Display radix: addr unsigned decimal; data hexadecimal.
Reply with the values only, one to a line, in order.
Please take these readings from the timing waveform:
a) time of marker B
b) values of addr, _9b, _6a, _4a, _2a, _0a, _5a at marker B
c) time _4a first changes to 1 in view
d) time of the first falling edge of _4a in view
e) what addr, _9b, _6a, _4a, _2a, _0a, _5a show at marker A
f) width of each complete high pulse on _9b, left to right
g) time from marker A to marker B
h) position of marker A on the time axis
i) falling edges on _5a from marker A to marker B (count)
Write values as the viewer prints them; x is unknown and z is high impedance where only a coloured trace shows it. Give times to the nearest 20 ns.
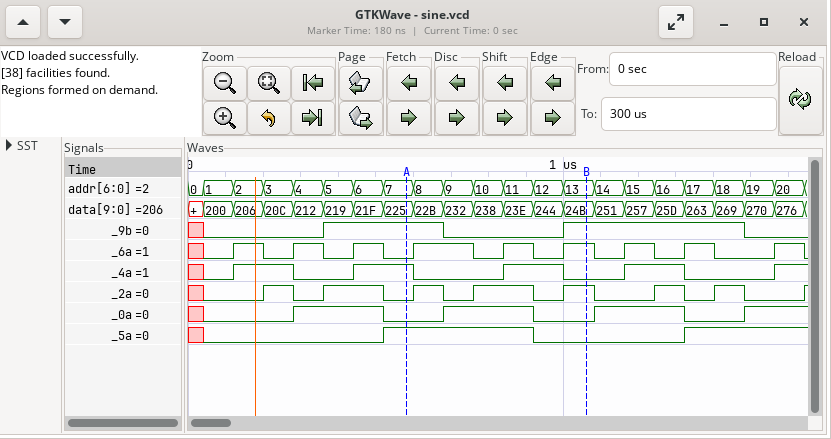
1060 ns
addr=13, _9b=1, _6a=1, _4a=0, _2a=1, _0a=0, _5a=0
120 ns
280 ns
addr=7, _9b=1, _6a=0, _4a=1, _2a=0, _0a=0, _5a=1
320 ns, 480 ns
480 ns
580 ns
1
